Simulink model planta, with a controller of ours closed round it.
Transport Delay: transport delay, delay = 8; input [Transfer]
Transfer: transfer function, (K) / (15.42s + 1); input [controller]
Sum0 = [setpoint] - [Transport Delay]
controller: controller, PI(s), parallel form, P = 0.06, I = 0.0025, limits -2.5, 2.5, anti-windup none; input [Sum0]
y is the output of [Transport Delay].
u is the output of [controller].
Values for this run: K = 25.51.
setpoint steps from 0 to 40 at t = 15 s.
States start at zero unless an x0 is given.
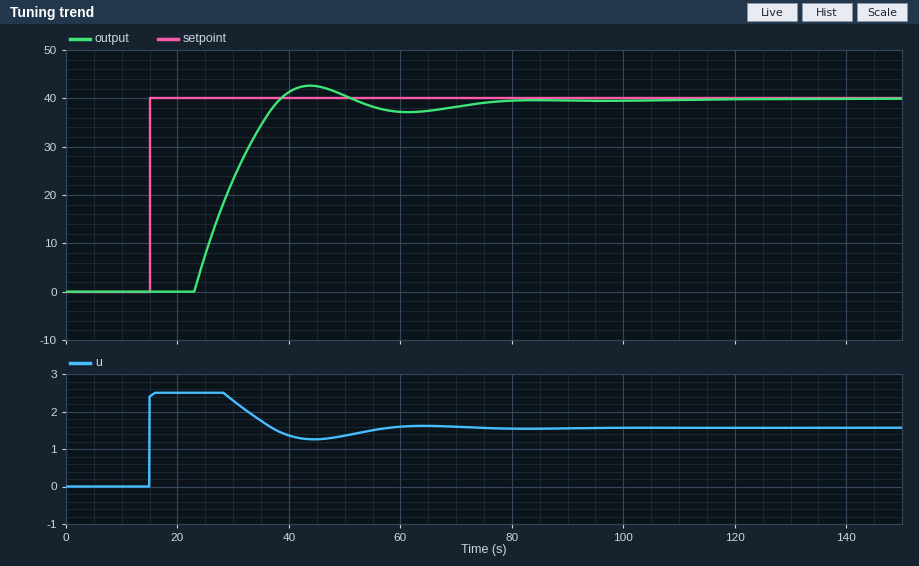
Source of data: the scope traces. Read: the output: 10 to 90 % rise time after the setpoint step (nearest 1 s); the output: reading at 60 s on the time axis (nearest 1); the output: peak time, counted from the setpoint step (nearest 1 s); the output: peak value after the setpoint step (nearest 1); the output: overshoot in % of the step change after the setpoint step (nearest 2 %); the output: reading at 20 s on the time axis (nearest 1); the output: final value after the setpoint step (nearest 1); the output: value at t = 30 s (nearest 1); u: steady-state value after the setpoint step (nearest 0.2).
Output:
12 s
37
29 s
43
6 %
0
40
23
1.6
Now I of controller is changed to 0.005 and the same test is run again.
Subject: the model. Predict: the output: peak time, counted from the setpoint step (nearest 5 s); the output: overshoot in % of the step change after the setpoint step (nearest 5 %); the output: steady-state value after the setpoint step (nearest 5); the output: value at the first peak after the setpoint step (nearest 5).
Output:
40 s
35 %
40
55
